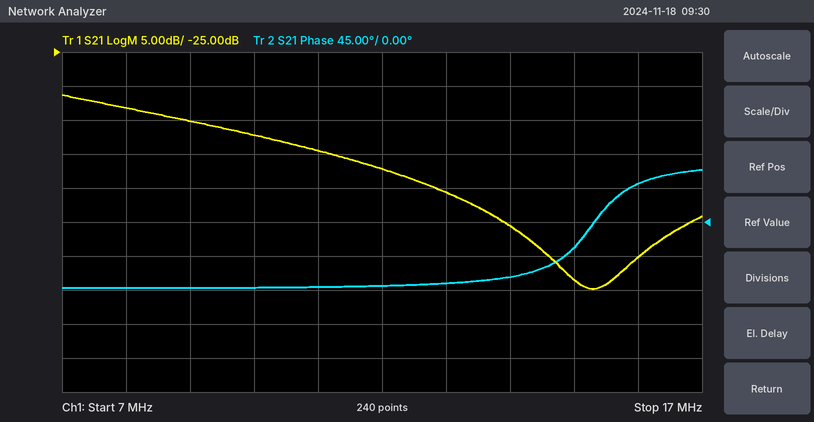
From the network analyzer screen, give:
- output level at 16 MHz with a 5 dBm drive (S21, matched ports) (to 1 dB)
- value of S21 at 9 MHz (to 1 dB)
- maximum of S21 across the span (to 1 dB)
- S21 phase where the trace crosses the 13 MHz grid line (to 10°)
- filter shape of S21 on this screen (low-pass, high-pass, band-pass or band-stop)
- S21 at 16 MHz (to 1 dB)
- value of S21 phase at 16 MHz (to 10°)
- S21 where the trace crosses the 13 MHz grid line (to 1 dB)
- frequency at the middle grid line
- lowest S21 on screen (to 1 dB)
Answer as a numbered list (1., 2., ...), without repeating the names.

1. -50 dBm
2. -35 dB
3. -31 dB
4. -80°
5. low-pass
6. -55 dB
7. 50°
8. -46 dB
9. 12 MHz
10. -60 dB
